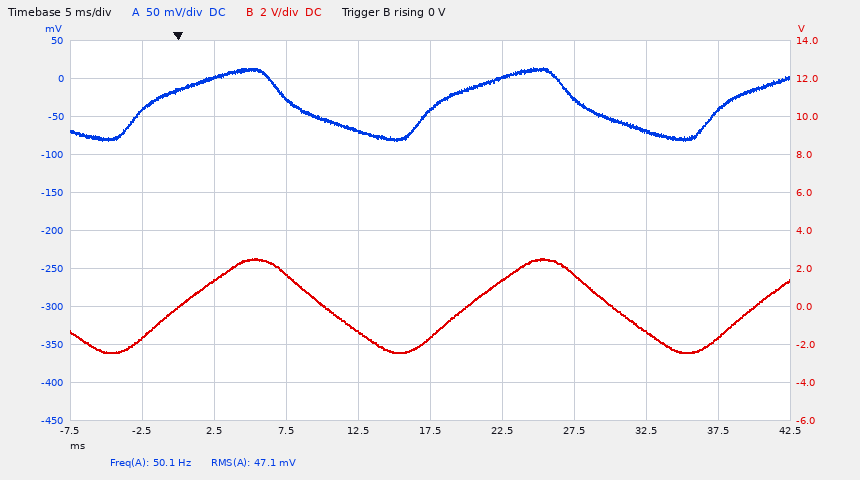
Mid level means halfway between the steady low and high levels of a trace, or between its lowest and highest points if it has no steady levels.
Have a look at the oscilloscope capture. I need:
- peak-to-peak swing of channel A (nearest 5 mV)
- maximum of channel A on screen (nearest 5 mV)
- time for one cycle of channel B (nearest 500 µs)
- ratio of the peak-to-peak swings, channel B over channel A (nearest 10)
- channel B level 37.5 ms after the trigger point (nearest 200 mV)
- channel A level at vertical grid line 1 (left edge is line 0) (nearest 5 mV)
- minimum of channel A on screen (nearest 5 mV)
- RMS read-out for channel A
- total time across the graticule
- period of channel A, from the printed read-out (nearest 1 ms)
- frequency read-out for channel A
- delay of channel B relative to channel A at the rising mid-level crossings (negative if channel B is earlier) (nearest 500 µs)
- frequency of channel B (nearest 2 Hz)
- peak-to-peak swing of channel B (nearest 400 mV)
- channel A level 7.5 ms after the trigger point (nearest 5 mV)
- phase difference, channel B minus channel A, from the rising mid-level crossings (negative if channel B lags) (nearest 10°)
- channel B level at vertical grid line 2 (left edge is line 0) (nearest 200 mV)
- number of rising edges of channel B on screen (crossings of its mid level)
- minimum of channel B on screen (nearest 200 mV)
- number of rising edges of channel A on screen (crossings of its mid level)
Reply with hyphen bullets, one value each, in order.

- 95 mV
- 15 mV
- 20.0 ms
- 50
- -1.6 V
- -40 mV
- -80 mV
- 47.1 mV
- 50 ms
- 20 ms
- 50.1 Hz
- +2.0 ms
- 50 Hz
- 4.8 V
- -25 mV
- -40°
- 1.4 V
- 3
- -2.4 V
- 3
